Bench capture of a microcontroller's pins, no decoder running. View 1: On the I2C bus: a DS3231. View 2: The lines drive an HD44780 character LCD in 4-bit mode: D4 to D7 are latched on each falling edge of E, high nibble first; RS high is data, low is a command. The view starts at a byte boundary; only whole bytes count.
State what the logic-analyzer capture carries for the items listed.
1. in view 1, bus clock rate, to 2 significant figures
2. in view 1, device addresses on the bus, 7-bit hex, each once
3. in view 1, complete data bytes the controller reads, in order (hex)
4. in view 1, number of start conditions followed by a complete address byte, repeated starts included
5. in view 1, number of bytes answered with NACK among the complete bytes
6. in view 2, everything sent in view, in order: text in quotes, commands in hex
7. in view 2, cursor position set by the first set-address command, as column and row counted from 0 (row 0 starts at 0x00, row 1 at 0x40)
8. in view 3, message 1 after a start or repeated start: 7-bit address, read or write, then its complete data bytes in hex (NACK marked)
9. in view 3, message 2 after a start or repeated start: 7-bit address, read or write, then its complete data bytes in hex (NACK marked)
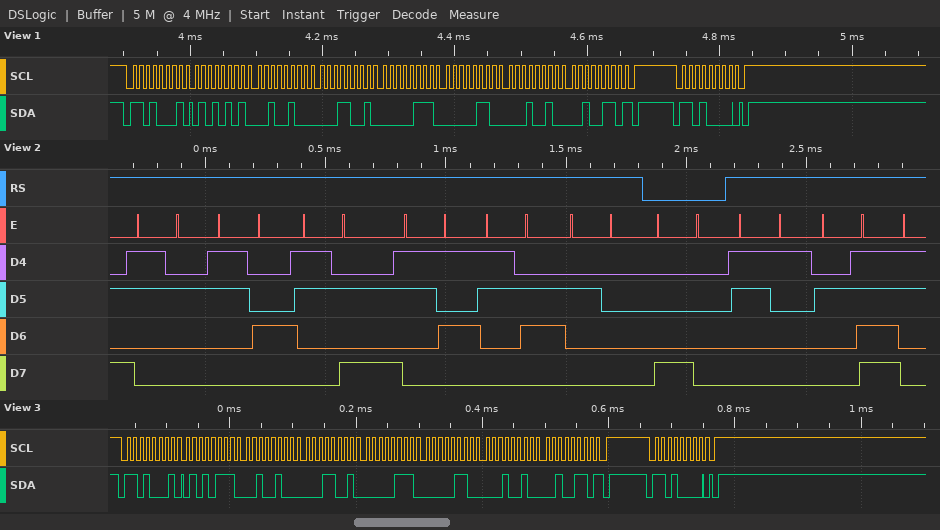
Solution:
100 kHz
0x68
55 24 19 07 06 12 26
2
1
"24:56 " 0x80 "1/"
column 0, row 0
0x68 read: 57 24 19 07 06 12 26 NACK
0x68 write
